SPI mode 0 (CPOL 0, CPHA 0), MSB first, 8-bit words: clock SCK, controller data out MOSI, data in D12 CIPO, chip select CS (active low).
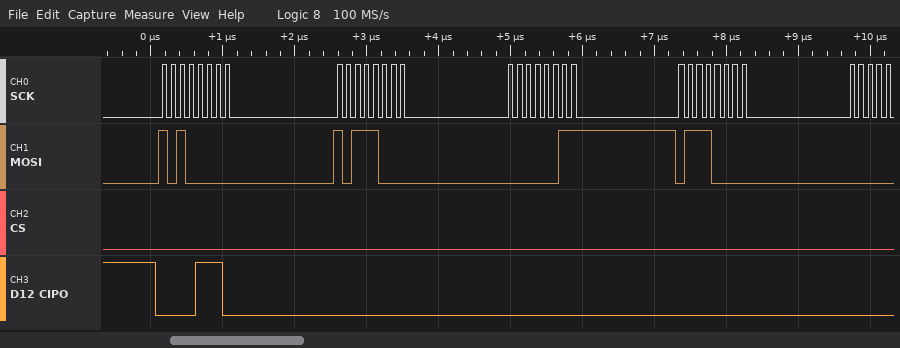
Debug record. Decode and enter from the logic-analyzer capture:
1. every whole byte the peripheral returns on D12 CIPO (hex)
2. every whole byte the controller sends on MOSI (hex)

0E 00 00 00
A0 B8 03 70
